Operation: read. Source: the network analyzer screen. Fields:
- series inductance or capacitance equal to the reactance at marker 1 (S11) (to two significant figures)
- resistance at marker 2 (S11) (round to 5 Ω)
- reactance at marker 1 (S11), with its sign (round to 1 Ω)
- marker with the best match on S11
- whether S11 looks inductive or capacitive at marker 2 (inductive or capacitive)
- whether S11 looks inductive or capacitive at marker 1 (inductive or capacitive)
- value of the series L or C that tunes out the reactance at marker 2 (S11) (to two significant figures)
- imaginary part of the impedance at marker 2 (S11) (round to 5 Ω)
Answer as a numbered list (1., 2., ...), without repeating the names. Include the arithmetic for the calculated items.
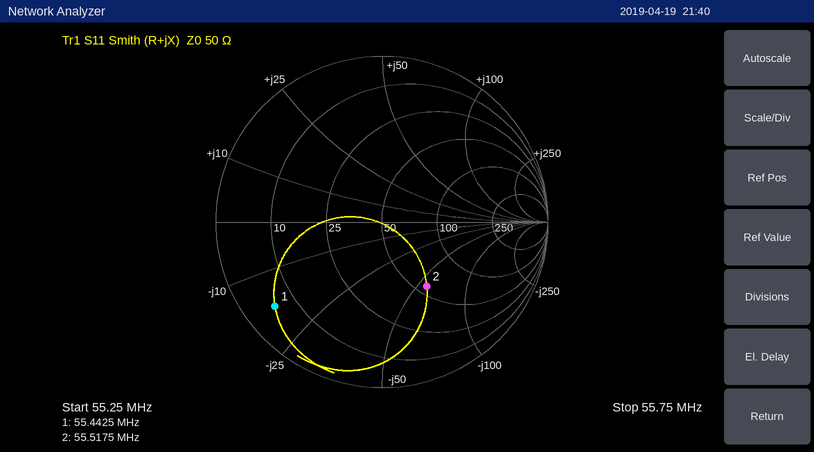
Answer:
1. C = 1/(2π × 55.4425 MHz × 17 Ω) ≈ 169 pF, so 170 pF to two significant figures
2. 55 Ω
3. -17 Ω
4. marker 2
5. capacitive
6. capacitive
7. L = 55 Ω/(2π × 55.5175 MHz) ≈ 158 nH, so 160 nH to two significant figures
8. -55 Ω
